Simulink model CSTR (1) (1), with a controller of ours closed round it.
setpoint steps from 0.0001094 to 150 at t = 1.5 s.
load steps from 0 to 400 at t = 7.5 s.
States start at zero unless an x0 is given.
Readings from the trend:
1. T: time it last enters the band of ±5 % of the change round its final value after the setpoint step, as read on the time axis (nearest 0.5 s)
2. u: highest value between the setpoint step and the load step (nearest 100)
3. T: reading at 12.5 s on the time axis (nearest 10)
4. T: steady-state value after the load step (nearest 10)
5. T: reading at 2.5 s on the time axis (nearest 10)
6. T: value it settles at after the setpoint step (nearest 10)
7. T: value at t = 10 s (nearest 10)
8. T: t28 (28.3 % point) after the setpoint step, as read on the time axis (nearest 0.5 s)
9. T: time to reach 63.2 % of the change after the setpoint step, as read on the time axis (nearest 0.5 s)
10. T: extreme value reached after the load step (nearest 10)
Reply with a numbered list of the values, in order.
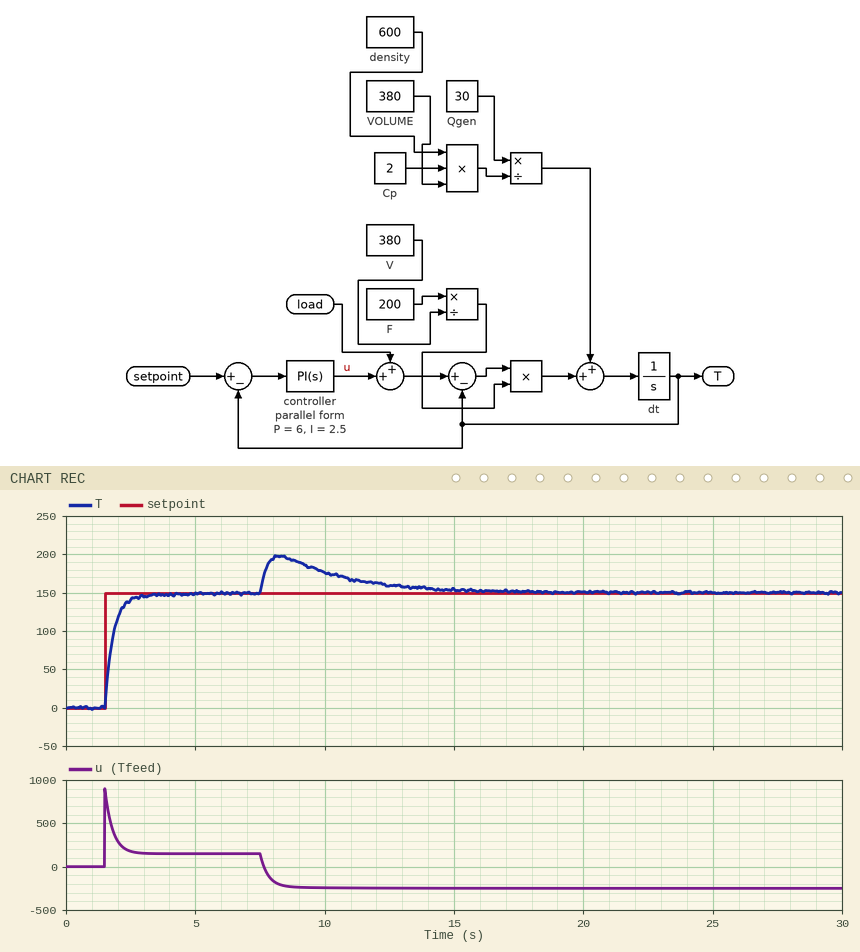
1. 2.5 s
2. 900
3. 160
4. 150
5. 140
6. 150
7. 180
8. 1.5 s
9. 2.0 s
10. 200
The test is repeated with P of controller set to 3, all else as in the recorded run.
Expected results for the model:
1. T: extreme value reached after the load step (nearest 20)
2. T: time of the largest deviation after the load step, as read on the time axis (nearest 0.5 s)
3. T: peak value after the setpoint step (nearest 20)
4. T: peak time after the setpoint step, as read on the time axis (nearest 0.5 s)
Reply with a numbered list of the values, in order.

1. 220
2. 8.5 s
3. 160
4. 4.0 s
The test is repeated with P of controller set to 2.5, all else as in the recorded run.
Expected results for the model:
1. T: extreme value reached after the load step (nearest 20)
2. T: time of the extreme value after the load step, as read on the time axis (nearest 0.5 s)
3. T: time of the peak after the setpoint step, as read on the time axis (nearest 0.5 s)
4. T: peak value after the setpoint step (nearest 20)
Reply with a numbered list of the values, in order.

1. 220
2. 8.5 s
3. 4.0 s
4. 160
